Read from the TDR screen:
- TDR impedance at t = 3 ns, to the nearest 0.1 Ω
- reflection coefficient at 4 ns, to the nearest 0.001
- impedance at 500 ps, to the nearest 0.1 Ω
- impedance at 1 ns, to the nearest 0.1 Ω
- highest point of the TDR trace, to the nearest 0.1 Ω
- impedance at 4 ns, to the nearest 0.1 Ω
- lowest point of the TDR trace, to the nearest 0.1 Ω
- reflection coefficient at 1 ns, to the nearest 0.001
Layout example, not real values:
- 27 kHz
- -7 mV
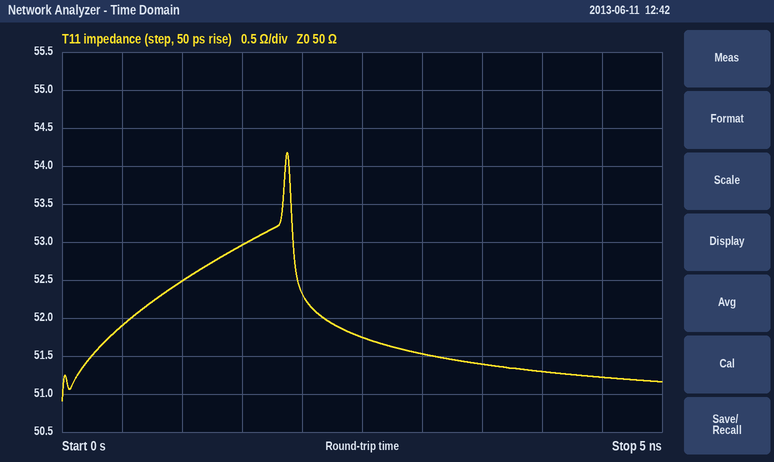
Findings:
- 51.5 Ω
- +0.013
- 51.9 Ω
- 52.5 Ω
- 54.2 Ω
- 51.3 Ω
- 50.9 Ω
- +0.024
